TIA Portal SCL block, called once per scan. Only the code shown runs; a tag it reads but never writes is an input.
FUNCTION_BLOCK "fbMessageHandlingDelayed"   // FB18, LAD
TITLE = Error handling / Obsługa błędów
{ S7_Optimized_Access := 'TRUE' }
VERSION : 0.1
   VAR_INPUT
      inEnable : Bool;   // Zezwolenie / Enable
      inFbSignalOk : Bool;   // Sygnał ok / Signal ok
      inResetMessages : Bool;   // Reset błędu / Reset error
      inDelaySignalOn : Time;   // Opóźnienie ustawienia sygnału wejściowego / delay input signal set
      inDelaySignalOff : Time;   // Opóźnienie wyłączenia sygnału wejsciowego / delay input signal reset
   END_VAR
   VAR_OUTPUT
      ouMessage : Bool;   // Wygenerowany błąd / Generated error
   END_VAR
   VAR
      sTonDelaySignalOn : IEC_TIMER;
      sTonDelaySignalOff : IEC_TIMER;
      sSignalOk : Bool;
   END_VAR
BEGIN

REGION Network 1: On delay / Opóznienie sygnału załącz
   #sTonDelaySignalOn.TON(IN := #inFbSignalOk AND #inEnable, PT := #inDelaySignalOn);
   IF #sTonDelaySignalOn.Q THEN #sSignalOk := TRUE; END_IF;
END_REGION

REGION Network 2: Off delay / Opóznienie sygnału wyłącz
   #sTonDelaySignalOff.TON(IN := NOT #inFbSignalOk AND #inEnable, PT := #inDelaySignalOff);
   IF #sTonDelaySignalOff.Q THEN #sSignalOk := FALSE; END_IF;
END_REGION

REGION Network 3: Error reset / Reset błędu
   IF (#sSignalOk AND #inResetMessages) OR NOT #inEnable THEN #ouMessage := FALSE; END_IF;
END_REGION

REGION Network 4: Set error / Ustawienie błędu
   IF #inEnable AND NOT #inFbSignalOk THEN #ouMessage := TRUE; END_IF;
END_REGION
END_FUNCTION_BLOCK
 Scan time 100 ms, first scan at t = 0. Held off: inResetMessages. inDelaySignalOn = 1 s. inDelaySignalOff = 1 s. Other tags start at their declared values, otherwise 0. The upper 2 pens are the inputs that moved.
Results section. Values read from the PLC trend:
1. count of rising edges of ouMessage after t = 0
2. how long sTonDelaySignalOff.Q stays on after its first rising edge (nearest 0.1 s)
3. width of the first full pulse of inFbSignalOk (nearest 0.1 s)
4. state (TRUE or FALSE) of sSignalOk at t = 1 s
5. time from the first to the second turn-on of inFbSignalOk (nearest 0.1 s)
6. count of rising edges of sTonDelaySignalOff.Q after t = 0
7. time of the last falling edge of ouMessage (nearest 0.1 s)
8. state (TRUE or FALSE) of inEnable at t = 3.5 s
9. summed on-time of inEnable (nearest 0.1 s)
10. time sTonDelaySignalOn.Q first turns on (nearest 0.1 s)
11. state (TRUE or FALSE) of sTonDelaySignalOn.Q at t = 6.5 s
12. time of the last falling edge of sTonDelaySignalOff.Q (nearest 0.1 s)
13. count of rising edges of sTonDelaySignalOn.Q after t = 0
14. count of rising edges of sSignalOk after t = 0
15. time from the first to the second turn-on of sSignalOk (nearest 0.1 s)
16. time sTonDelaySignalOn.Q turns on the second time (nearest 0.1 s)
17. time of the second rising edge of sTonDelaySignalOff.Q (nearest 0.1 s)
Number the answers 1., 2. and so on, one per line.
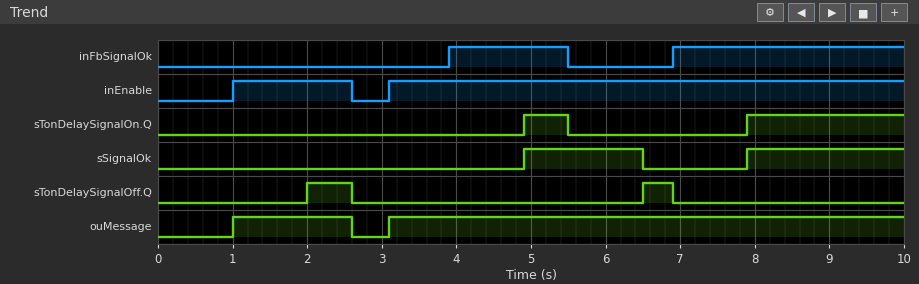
1. 2
2. 0.6 s
3. 1.6 s
4. FALSE
5. 3.0 s
6. 2
7. 2.6 s
8. TRUE
9. 8.5 s
10. 4.9 s
11. FALSE
12. 6.9 s
13. 2
14. 2
15. 3.0 s
16. 7.9 s
17. 6.5 s
